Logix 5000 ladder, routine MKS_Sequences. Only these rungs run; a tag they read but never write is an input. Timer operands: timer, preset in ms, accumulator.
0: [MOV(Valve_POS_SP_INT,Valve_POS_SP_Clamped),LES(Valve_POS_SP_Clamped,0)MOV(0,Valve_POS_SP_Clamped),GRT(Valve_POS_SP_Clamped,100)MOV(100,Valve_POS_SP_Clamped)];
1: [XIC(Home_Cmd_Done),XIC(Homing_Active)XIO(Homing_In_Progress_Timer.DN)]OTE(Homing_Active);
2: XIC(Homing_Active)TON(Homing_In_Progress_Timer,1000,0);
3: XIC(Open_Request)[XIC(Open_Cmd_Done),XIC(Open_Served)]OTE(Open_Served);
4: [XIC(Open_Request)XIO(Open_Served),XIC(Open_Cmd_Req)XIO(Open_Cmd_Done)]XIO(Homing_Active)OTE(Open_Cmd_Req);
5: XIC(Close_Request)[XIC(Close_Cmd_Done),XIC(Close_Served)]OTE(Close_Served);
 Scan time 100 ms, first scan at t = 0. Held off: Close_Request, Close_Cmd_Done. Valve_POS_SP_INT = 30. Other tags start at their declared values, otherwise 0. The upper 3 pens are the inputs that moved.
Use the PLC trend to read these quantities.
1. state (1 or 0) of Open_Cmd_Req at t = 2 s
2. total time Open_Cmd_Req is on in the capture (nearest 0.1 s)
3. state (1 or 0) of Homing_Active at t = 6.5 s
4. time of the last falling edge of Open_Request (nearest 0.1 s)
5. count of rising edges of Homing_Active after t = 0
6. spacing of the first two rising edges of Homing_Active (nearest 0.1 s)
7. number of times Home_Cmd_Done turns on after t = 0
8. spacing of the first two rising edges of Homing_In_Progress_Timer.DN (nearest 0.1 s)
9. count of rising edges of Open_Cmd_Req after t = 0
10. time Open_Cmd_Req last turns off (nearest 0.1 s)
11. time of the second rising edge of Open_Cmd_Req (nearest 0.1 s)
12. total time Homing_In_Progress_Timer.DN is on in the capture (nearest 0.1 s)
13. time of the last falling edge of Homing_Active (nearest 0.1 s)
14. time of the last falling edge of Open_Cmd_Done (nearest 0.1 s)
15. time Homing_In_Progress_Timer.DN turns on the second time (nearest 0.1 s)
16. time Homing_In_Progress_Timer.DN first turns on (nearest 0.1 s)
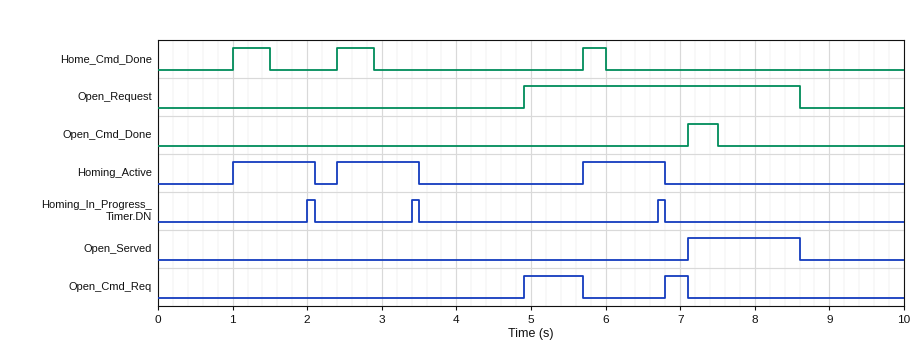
0
1.1 s
1
8.6 s
3
1.4 s
3
1.4 s
2
7.1 s
6.8 s
0.3 s
6.8 s
7.5 s
3.4 s
2.0 s
